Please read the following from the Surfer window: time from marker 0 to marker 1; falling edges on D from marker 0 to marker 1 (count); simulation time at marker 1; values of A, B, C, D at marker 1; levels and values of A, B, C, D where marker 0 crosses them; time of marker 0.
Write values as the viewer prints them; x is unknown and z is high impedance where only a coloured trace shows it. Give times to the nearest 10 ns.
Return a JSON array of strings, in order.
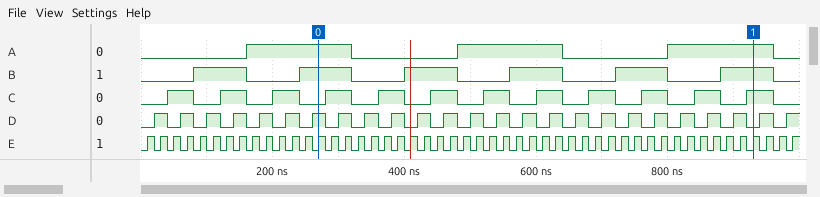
["660 ns", "17", "930 ns", "A=1, B=1, C=1, D=0", "A=1, B=1, C=0, D=1", "270 ns"]
